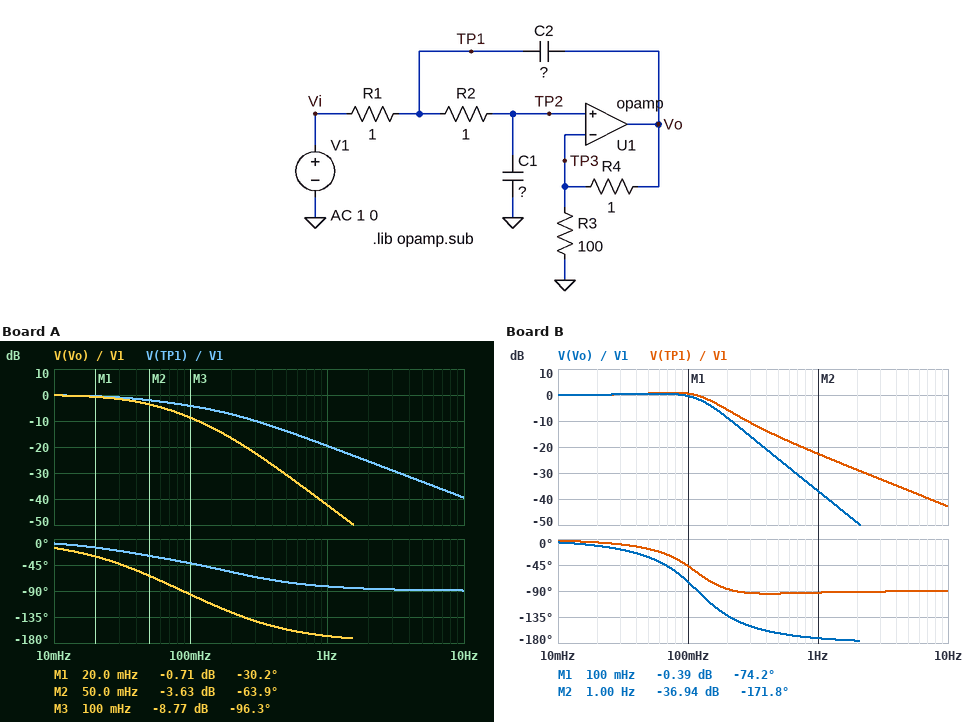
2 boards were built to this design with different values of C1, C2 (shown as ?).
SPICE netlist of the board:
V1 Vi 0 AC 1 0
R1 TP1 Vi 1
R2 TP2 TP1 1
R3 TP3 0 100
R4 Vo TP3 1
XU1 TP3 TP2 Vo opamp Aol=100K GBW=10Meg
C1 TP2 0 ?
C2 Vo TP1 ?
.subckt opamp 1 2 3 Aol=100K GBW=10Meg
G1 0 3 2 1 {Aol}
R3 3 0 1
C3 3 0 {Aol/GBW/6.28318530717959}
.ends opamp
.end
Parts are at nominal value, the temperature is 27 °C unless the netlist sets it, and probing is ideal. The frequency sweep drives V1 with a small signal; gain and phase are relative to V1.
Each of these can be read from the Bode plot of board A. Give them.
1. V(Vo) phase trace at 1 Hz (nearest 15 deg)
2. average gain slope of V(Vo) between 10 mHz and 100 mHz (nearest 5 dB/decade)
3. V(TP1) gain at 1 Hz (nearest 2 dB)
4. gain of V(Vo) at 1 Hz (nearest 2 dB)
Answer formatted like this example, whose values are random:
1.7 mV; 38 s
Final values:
-165 deg; -10 dB/decade; -20 dB; -42 dB
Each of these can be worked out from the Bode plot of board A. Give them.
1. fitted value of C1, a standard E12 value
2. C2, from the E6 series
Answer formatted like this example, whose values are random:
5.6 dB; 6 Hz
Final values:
2.2 F; 1.5 F
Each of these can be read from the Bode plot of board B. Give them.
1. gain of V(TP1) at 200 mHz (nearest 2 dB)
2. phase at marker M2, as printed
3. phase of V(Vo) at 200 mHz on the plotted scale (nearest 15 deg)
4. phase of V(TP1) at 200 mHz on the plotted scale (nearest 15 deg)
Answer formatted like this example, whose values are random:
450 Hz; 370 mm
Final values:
-6 dB; -171.8 deg; -135 deg; -90 deg
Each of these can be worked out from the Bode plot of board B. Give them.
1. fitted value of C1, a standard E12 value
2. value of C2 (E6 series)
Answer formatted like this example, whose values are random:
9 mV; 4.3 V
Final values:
820 mF; 2.2 F
